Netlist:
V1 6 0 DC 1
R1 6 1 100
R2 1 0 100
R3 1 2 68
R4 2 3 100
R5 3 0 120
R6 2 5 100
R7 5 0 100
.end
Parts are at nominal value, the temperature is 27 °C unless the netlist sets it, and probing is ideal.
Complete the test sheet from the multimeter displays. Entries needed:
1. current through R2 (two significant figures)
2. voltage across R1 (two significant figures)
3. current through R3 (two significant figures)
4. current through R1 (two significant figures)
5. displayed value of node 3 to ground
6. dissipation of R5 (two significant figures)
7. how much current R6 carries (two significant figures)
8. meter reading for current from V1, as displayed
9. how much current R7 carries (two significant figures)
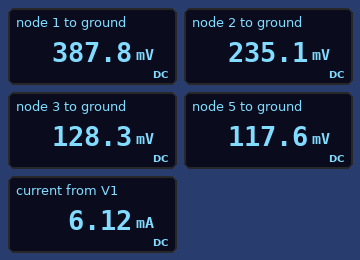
3.9 mA
610 mV
2.2 mA
6.1 mA
128.3 mV
140 µW
1.2 mA
6.12 mA
1.2 mA
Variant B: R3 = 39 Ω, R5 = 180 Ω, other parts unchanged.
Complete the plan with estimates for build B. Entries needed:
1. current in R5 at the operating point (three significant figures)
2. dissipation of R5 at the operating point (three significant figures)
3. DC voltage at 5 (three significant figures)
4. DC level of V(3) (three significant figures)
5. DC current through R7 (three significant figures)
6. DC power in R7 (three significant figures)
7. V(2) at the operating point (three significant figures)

1.01 mA
185 µW
142 mV
182 mV
1.42 mA
201 µW
284 mV
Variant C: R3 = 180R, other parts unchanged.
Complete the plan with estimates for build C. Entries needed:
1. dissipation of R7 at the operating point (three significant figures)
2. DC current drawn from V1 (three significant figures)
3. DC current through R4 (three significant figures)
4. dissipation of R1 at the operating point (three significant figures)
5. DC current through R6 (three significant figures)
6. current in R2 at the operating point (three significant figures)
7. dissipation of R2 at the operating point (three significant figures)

61.2 µW
5.75 mA
711 µA
3.30 mW
782 µA
4.25 mA
1.81 mW
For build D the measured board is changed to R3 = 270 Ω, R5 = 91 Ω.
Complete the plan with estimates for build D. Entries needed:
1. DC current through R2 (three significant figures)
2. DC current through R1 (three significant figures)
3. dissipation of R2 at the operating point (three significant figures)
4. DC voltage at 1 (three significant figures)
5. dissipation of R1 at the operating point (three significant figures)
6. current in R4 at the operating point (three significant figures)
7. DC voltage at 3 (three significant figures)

4.40 mA
5.60 mA
1.94 mW
440 mV
3.13 mW
612 µA
55.7 mV
